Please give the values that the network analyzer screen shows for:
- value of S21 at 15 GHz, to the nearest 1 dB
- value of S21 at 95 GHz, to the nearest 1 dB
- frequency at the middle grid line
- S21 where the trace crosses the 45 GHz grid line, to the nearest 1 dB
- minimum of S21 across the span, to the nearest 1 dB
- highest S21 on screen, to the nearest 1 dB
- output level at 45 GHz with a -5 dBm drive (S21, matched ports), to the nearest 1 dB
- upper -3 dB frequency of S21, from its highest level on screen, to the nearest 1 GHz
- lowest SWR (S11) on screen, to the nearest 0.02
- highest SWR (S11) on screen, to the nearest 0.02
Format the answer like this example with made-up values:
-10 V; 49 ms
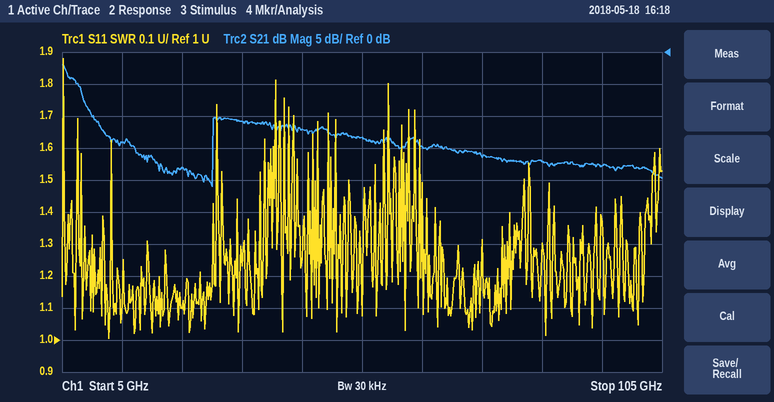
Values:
-14 dB; -18 dB; 55 GHz; -12 dB; -21 dB; -2 dB; -17 dBm; 8 GHz; 1.00; 1.88
